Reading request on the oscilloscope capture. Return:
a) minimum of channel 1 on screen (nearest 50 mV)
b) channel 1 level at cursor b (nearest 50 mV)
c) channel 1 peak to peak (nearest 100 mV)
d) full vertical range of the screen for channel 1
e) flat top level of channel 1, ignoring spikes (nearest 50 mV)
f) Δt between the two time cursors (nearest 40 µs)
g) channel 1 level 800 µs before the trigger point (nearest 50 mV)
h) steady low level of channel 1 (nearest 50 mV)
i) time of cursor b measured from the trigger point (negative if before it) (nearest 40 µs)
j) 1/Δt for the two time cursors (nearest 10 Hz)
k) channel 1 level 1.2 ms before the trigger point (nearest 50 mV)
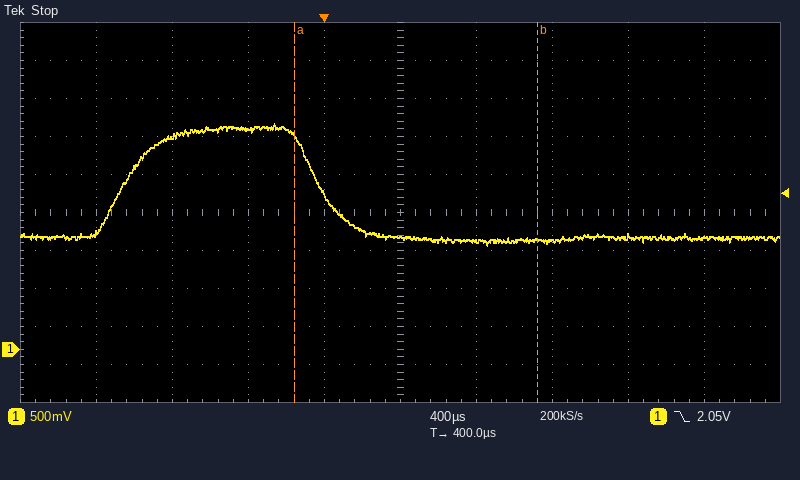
1.35 V
1.45 V
1.60 V
5 V
2.90 V
1.28 ms
2.80 V
1.45 V
+1.12 ms
780 Hz
1.55 V
